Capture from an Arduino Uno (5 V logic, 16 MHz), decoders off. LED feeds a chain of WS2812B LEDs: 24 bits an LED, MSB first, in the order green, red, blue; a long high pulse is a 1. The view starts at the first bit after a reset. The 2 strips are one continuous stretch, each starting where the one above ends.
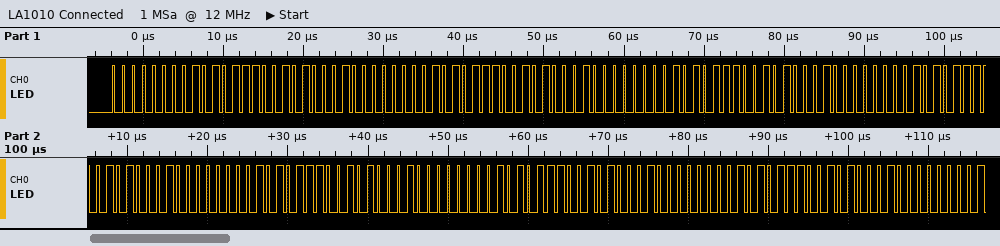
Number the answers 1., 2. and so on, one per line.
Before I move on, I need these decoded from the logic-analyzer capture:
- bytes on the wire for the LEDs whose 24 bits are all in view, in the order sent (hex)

1. 00 AE 51 00 AE 51 00 AE 51 00 AE 51 00 AE 51 00 AE 51 00 AE 51
